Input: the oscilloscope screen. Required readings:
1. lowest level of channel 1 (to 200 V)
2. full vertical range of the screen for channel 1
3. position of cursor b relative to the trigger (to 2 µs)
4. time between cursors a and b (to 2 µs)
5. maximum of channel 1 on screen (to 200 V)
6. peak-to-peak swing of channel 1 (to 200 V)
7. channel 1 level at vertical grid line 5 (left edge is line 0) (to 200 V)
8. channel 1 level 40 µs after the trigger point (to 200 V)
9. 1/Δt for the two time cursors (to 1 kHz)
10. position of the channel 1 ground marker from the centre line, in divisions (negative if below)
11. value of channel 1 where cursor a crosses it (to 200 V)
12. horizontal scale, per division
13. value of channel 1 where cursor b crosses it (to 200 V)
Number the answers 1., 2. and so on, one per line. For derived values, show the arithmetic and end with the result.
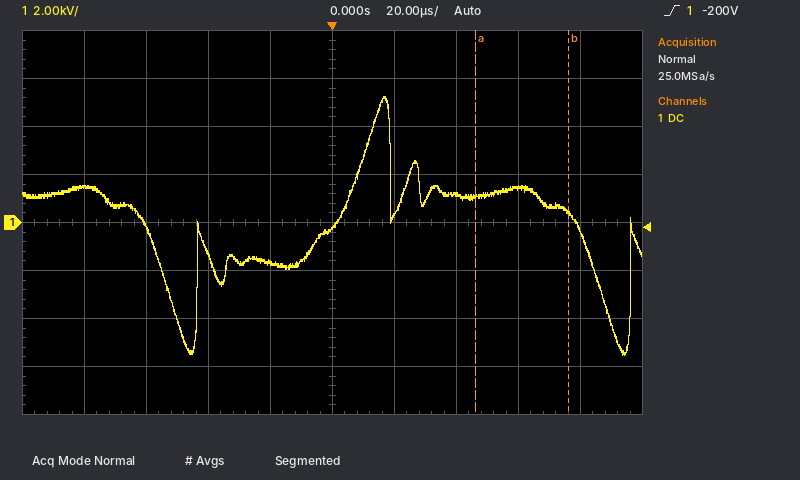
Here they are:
1. -5.6 kV
2. 16 kV
3. +76 µs
4. 30 µs
5. 5.2 kV
6. 5.2 kV − (-5.6 kV) = 10.8 kV
7. -200 V
8. 1.2 kV
9. 1 / 30 µs ≈ 33 kHz
10. 0.0 div
11. 1.0 kV
12. 20 µs
13. 400 V
